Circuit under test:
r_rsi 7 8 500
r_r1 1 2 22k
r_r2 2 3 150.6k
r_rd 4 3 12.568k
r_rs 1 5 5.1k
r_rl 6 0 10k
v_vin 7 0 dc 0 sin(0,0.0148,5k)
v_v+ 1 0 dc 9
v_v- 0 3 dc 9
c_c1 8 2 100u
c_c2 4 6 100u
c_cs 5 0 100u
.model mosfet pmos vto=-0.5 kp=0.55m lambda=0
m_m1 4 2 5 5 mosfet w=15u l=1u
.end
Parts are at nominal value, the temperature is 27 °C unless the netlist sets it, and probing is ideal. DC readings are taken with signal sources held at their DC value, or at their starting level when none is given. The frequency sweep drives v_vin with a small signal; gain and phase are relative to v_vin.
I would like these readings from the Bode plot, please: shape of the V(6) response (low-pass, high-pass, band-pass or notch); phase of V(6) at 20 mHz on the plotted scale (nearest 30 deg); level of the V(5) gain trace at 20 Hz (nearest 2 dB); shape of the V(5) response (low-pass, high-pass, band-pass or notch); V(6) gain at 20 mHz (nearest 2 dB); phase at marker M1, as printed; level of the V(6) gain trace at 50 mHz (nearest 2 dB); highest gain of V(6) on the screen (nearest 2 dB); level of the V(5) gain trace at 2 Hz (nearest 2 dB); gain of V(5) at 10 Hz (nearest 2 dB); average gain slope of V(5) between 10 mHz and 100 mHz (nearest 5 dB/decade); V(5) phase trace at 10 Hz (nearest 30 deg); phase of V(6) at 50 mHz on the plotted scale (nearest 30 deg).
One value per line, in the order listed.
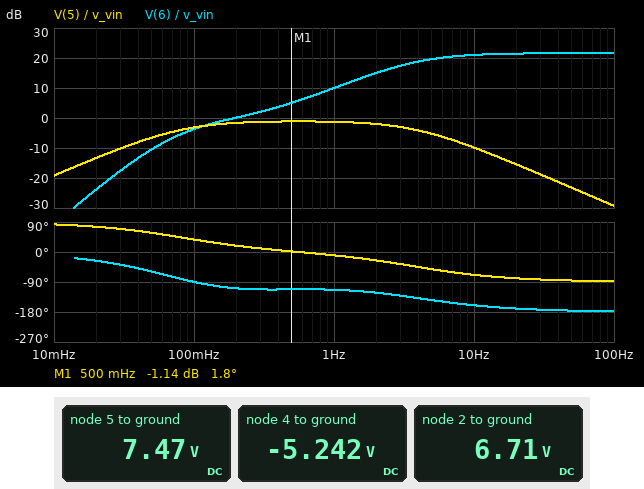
high-pass
-30 deg
-16 dB
band-pass
-24 dB
1.8 deg
-10 dB
22 dB
-2 dB
-10 dB
15 dB/decade
-60 deg
-60 deg
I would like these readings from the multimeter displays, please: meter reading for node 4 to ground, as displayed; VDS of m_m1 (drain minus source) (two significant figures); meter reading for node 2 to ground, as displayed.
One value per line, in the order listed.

-5.242 V
-13 V
6.71 V
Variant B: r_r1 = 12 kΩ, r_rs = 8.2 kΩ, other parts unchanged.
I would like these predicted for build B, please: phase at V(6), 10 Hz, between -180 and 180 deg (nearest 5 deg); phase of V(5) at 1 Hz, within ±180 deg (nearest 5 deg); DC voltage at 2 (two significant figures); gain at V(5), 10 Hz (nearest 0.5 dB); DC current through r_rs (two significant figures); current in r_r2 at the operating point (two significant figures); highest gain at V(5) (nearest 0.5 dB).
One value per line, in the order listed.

-170 deg
-20 deg
7.7 V
-15.0 dB
84 µA
110 µA
-2.0 dB
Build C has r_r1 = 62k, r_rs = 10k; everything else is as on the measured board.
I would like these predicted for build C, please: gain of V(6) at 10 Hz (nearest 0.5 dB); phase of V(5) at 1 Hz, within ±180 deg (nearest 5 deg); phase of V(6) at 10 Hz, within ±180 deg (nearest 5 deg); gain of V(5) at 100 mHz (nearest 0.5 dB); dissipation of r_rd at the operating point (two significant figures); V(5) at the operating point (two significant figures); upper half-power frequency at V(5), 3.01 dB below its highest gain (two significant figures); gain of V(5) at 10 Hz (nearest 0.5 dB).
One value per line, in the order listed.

22.5 dB
-10 deg
-155 deg
-1.0 dB
2.5 mW
4.6 V
4.5 Hz
-8.0 dB
